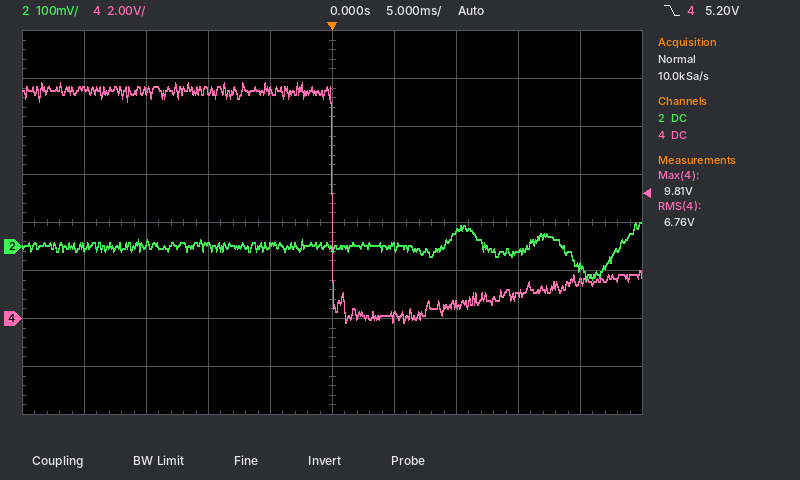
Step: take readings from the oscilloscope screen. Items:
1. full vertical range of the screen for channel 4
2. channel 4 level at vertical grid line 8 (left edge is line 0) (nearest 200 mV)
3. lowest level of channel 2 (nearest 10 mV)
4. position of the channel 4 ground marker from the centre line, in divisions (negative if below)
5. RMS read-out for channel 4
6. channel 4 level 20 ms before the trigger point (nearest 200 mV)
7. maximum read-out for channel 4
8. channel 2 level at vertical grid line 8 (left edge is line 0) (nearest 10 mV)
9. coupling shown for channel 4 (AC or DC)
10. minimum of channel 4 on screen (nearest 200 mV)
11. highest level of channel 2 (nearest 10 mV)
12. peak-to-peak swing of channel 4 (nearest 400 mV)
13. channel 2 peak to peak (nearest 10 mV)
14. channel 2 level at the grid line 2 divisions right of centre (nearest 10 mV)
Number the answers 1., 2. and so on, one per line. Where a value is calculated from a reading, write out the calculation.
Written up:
1. 16 V
2. 1.0 V
3. -70 mV
4. -2.0 div
5. 6.76 V
6. 9.6 V
7. 9.81 V
8. -10 mV
9. DC
10. -200 mV
11. 50 mV
12. 10.0 V
13. 50 mV − (-70 mV) = 120 mV
14. 30 mV
